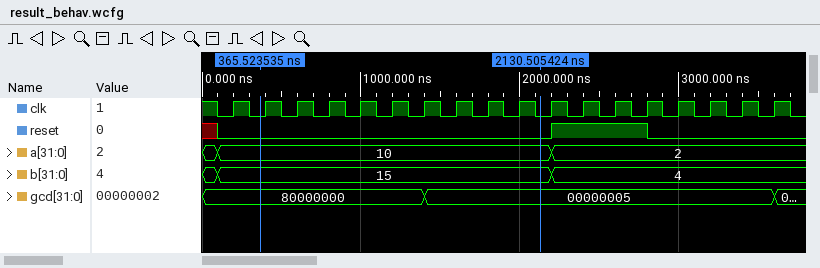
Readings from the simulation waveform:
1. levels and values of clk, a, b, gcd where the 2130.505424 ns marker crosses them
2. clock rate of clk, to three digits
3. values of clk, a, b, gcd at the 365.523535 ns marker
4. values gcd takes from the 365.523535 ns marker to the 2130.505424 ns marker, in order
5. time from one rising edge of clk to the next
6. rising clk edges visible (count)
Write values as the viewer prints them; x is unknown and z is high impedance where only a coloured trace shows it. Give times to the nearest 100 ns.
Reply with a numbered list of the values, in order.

1. clk=0, a=10, b=15, gcd=00000005
2. 5.00 MHz
3. clk=0, a=10, b=15, gcd=80000000
4. 80000000, 00000005
5. 200 ns
6. 18
